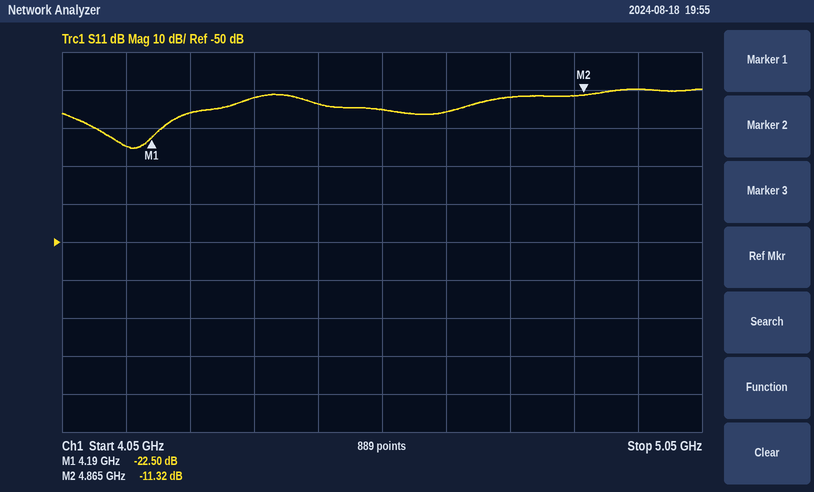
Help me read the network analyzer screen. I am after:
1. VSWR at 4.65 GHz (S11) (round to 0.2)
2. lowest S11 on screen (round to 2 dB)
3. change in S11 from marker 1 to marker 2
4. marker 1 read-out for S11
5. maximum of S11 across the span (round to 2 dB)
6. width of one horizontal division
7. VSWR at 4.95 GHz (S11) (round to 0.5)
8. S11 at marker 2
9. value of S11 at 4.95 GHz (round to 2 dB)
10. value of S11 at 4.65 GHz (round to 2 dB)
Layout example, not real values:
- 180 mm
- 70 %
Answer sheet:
- 1.4
- -26 dB
- 11.18 dB
- -22.50 dB
- -10 dB
- 100 MHz
- 2.0
- -11.32 dB
- -10 dB
- -16 dB
